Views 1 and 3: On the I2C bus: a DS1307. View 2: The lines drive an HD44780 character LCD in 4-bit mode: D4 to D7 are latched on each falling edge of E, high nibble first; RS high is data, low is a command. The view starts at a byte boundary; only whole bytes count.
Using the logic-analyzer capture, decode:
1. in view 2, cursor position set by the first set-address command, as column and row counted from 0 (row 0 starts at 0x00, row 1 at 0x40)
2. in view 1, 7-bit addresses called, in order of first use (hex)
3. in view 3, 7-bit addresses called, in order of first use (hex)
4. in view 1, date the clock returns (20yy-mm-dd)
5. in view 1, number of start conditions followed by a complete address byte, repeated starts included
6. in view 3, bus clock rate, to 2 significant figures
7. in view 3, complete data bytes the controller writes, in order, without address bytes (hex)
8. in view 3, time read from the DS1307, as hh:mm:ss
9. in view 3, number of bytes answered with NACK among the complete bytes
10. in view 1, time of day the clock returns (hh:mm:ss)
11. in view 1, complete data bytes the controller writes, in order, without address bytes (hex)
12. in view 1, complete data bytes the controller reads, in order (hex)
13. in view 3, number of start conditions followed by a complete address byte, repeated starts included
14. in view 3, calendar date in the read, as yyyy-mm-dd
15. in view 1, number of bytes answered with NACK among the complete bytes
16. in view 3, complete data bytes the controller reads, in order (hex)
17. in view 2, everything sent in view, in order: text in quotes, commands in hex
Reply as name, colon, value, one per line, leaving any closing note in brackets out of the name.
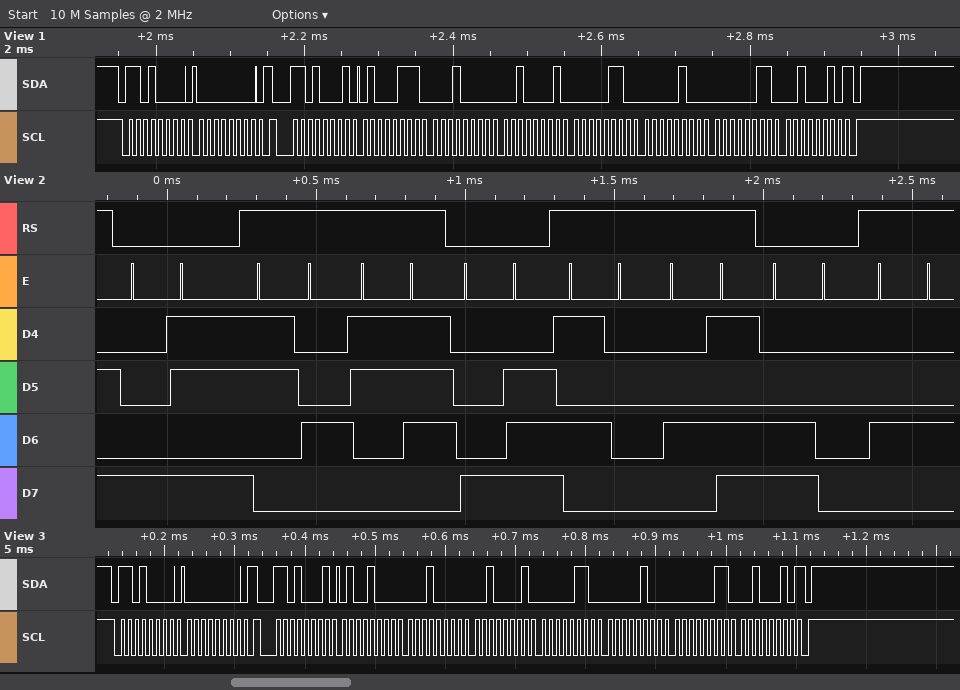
in view 2, cursor position set by the first set-address command, as column and row counted from 0: column 11, row 0
in view 1, 7-bit addresses called, in order of first use: 0x68
in view 3, 7-bit addresses called, in order of first use: 0x68
in view 1, date the clock returns: 2022-03-04
in view 1, number of start conditions followed by a complete address byte, repeated starts included: 2
in view 3, bus clock rate, to 2 significant figures: 100 kHz
in view 3, complete data bytes the controller writes, in order, without address bytes: 00
in view 3, time read from the DS1307, as hh:mm:ss: 21:10:48
in view 3, number of bytes answered with NACK among the complete bytes: 1
in view 1, time of day the clock returns: 21:10:47
in view 1, complete data bytes the controller writes, in order, without address bytes: 00
in view 1, complete data bytes the controller reads, in order: 47 10 21 06 04 03 22
in view 3, number of start conditions followed by a complete address byte, repeated starts included: 2
in view 3, calendar date in the read, as yyyy-mm-dd: 2022-03-04
in view 1, number of bytes answered with NACK among the complete bytes: 1
in view 3, complete data bytes the controller reads, in order: 48 10 21 06 04 03 22
in view 2, everything sent in view, in order: text in quotes, commands in hex: 0x8B "47" 0x8E "PM" 0xC0 "D"
